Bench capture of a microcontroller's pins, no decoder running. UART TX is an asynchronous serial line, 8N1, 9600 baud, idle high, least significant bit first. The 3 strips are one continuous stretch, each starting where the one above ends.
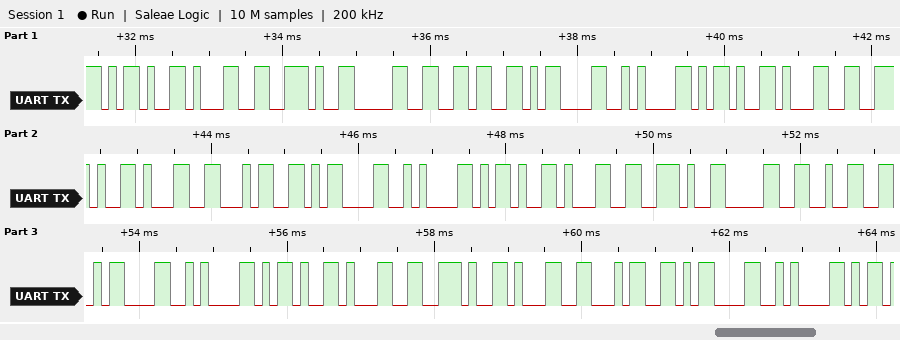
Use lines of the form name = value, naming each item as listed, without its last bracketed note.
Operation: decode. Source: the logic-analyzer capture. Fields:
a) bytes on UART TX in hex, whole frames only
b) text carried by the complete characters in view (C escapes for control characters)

bytes on UART TX in hex, whole frames only = 0x2D 0x31 0x2E 0x30 0x36 0x0D 0x0A 0x2D 0x31 0x2E 0x31 0x34 0x0D 0x0A 0x2D 0x31 0x2E 0x30 0x32 0x0D 0x0A 0x2D 0x31 0x2E 0x31 0x34 0x0D 0x0A
text carried by the complete characters in view = "-1.06\r\n-1.14\r\n-1.02\r\n-1.14\r\n"
